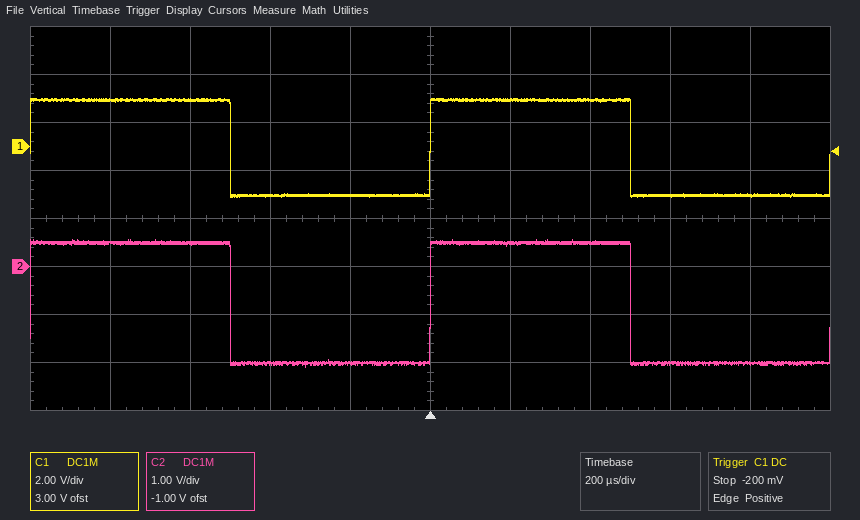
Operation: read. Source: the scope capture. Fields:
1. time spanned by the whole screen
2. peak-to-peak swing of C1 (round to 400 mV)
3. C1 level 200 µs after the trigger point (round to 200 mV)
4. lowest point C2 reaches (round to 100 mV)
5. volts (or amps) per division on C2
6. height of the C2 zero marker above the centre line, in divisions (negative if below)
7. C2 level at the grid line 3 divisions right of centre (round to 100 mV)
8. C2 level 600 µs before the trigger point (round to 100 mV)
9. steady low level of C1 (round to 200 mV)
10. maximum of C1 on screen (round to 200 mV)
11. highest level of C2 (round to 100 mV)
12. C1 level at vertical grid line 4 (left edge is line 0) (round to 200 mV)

2 ms
4.0 V
2.0 V
-2.1 V
1 V
-1.0 div
-2.0 V
500 mV
-2.0 V
2.0 V
600 mV
-2.0 V
